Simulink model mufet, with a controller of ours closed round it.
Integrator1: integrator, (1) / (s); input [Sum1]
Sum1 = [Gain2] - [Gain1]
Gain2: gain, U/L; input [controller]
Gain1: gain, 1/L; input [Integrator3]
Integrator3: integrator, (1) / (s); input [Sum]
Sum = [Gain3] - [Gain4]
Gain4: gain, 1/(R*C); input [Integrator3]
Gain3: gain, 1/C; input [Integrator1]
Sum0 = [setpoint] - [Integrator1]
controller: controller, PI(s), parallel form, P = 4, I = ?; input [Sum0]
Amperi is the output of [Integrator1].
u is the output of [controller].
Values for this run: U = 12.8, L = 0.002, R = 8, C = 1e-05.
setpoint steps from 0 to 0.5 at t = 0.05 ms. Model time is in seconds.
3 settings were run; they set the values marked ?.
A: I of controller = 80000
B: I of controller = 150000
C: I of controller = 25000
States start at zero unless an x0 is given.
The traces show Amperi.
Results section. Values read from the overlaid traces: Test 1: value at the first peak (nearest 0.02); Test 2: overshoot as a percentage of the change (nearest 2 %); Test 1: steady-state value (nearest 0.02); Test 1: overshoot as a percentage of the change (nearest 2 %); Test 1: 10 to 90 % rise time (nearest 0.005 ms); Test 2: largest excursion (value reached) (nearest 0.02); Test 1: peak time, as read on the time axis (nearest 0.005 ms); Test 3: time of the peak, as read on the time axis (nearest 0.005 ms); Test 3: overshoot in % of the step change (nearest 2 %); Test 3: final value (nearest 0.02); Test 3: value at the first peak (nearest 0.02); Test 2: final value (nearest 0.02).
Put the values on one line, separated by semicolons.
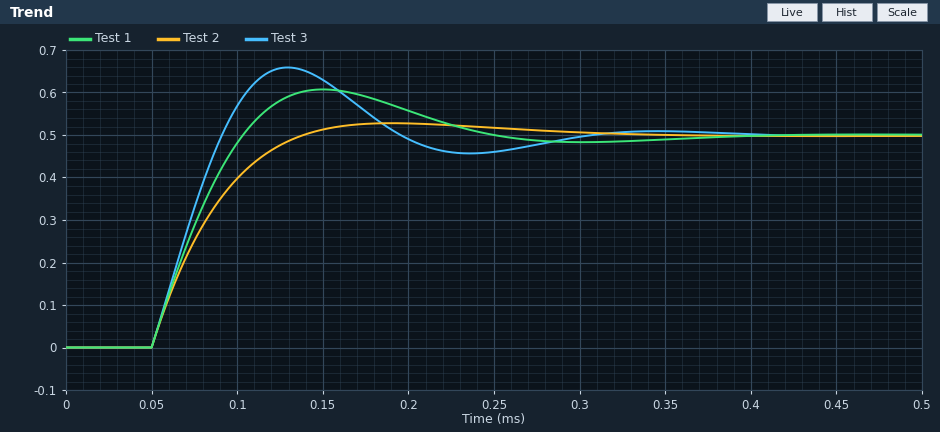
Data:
0.60; 6 %; 0.50; 22 %; 0.040 ms; 0.52; 0.150 ms; 0.130 ms; 32 %; 0.50; 0.66; 0.50
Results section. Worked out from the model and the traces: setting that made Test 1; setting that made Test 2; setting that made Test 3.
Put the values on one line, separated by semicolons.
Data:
A; C; B
